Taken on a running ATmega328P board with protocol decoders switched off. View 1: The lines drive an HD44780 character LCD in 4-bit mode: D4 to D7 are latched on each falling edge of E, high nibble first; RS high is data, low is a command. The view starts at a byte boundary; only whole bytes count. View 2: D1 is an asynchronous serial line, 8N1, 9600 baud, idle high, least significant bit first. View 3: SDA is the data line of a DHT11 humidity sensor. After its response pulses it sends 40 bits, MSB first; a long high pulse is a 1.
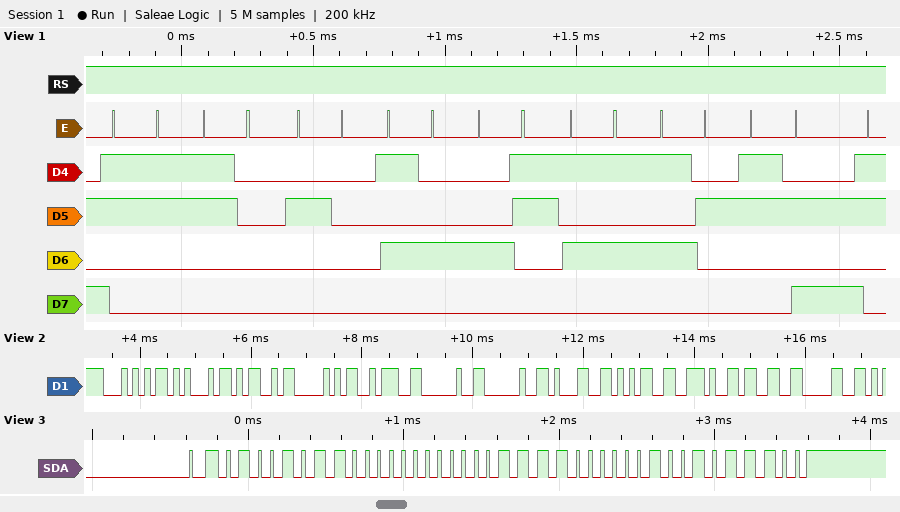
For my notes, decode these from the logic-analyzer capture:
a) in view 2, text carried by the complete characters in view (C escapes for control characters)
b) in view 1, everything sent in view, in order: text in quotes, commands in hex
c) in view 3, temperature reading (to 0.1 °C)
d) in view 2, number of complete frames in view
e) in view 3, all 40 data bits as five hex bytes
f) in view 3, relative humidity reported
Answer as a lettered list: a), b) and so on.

a) "TEMP:  15.30"
b) "30 TCUR:"
c) 15.2 °C
d) 12
e) 4B 00 0F 02 5C
f) 75 %
